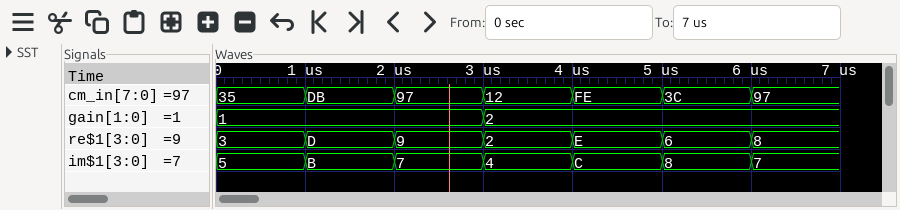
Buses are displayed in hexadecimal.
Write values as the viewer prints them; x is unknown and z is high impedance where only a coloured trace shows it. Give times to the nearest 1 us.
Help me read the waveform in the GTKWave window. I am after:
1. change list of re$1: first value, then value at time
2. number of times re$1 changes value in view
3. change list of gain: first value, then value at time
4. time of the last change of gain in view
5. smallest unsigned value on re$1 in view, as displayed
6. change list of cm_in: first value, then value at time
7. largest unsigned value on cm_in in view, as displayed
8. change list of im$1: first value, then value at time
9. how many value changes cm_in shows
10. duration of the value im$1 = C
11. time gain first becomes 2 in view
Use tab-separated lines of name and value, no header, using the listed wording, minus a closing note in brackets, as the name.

change list of re$1: first value, then value at time	3, D at 1 us, 9 at 2 us, 2 at 3 us, E at 4 us, 6 at 5 us, 8 at 6 us
number of times re$1 changes value in view	6
change list of gain: first value, then value at time	1, 2 at 3 us
time of the last change of gain in view	3 us
smallest unsigned value on re$1 in view, as displayed	2
change list of cm_in: first value, then value at time	35, DB at 1 us, 97 at 2 us, 12 at 3 us, FE at 4 us, 3C at 5 us, 97 at 6 us
largest unsigned value on cm_in in view, as displayed	FE
change list of im$1: first value, then value at time	5, B at 1 us, 7 at 2 us, 4 at 3 us, C at 4 us, 8 at 5 us, 7 at 6 us
how many value changes cm_in shows	6
duration of the value im$1 = C	1 us
time gain first becomes 2 in view	3 us
